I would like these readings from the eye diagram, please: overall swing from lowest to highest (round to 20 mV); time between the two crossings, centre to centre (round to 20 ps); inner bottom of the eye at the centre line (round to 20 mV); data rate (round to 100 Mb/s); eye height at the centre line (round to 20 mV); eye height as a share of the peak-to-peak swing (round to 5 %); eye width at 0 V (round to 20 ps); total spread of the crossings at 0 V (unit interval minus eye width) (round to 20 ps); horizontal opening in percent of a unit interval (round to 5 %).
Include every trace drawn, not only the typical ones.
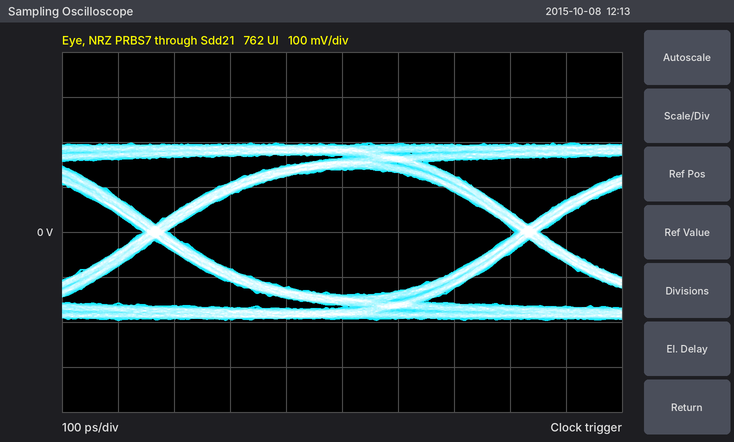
400 mV
660 ps
-140 mV
1.5 Gb/s
280 mV
70 %
620 ps
40 ps
95 %
